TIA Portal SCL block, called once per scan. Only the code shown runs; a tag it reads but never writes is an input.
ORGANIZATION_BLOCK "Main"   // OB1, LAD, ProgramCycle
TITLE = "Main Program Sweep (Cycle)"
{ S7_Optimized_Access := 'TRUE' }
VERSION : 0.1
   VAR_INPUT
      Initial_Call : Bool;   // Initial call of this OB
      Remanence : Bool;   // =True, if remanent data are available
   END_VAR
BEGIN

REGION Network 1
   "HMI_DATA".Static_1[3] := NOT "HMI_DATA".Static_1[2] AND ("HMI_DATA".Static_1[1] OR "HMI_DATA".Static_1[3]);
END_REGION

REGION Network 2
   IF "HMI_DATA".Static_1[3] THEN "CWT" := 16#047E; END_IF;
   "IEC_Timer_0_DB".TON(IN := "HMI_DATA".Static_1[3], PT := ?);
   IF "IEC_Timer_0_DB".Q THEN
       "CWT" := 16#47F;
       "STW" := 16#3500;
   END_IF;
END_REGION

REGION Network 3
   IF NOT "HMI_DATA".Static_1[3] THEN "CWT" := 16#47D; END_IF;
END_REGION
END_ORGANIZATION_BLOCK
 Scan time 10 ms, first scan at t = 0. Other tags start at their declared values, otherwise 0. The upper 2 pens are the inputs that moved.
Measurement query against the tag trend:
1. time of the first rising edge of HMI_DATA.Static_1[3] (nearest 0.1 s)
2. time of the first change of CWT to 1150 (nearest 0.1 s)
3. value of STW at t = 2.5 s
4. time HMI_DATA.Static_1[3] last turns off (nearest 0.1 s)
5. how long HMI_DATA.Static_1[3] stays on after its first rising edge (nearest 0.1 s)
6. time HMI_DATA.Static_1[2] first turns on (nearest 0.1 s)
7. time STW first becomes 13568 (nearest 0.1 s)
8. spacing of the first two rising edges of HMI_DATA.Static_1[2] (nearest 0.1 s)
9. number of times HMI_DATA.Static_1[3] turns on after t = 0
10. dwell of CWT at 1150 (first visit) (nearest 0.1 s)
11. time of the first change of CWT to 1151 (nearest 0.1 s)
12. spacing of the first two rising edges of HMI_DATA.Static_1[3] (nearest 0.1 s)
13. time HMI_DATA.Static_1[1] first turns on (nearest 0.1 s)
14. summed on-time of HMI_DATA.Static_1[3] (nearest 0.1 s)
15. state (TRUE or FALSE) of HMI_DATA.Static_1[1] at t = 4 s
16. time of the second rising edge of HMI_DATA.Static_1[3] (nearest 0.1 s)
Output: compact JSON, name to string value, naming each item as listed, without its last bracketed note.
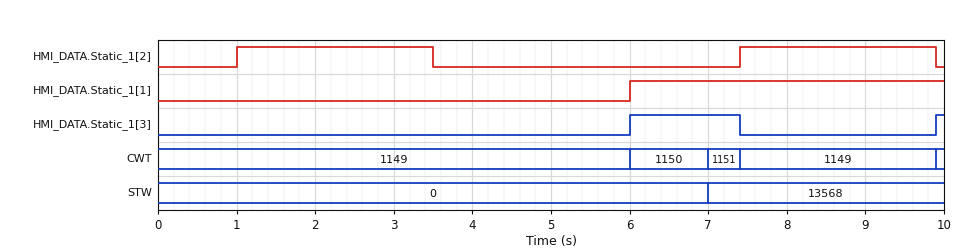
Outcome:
{"time of the first rising edge of HMI_DATA.Static_1[3]": "6.0 s", "time of the first change of CWT to 1150": "6.0 s", "value of STW at t = 2.5 s": "0", "time HMI_DATA.Static_1[3] last turns off": "7.4 s", "how long HMI_DATA.Static_1[3] stays on after its first rising edge": "1.4 s", "time HMI_DATA.Static_1[2] first turns on": "1.0 s", "time STW first becomes 13568": "7.0 s", "spacing of the first two rising edges of HMI_DATA.Static_1[2]": "6.4 s", "number of times HMI_DATA.Static_1[3] turns on after t = 0": "2", "dwell of CWT at 1150 (first visit)": "1.0 s", "time of the first change of CWT to 1151": "7.0 s", "spacing of the first two rising edges of HMI_DATA.Static_1[3]": "3.9 s", "time HMI_DATA.Static_1[1] first turns on": "6.0 s", "summed on-time of HMI_DATA.Static_1[3]": "1.5 s", "state (TRUE or FALSE) of HMI_DATA.Static_1[1] at t = 4 s": "FALSE", "time of the second rising edge of HMI_DATA.Static_1[3]": "9.9 s"}
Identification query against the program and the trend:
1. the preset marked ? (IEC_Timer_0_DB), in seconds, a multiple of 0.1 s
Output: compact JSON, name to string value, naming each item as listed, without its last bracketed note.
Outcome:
{"the preset marked ? (IEC_Timer_0_DB), in seconds, a multiple of 0.1 s": "1.0 s"}
